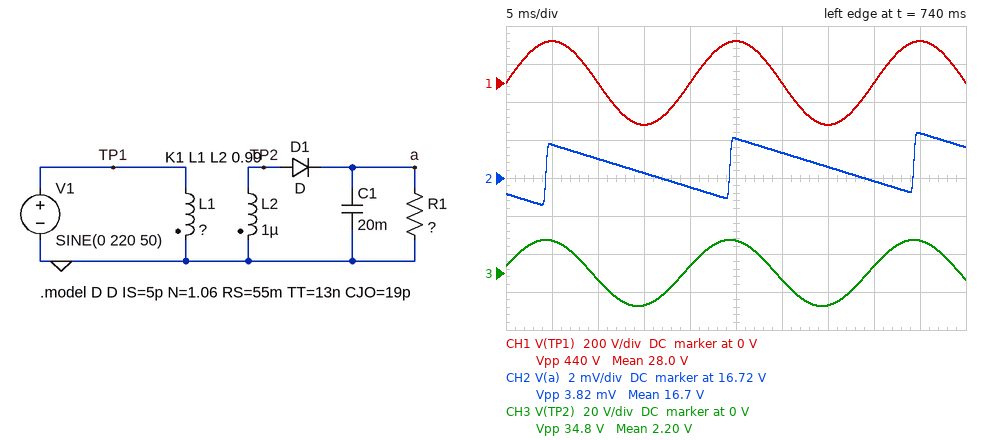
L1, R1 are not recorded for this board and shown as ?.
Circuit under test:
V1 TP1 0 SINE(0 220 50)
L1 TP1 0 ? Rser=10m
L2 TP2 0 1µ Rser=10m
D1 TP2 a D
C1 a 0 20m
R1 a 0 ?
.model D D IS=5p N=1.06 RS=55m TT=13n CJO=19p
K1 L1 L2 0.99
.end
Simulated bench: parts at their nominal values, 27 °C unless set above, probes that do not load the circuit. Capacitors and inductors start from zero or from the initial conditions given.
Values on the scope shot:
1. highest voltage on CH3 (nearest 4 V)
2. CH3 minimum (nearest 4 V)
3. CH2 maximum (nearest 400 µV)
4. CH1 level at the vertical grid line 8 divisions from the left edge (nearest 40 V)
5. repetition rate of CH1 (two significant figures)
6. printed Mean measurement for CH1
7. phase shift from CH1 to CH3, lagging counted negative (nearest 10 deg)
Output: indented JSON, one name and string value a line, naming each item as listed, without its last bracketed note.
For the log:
{
  "highest voltage on CH3": "16 V",
  "CH3 minimum": "-16 V",
  "CH2 maximum": "16.7184 V",
  "CH1 level at the vertical grid line 8 divisions from the left edge": "0 V",
  "repetition rate of CH1": "50 Hz",
  "printed Mean measurement for CH1": "28.0 V",
  "phase shift from CH1 to CH3, lagging counted negative": "10 deg"
}
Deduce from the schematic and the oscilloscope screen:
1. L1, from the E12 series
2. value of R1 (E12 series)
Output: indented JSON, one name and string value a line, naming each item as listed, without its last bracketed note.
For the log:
{
  "L1, from the E12 series": "150 µH",
  "value of R1": "5.6 kΩ"
}
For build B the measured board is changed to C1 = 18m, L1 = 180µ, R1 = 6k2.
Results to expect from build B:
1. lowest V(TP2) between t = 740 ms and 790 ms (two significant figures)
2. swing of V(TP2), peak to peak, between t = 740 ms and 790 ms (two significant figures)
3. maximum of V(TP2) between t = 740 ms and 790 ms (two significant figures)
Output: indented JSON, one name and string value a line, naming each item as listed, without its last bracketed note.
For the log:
{
  "lowest V(TP2) between t = 740 ms and 790 ms": "-16 V",
  "swing of V(TP2), peak to peak, between t = 740 ms and 790 ms": "32 V",
  "maximum of V(TP2) between t = 740 ms and 790 ms": "16 V"
}
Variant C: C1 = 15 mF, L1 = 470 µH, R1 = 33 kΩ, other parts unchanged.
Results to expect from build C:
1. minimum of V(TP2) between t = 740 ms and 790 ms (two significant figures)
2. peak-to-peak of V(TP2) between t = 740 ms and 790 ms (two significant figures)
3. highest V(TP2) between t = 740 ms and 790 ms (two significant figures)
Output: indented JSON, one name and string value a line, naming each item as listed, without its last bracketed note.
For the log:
{
  "minimum of V(TP2) between t = 740 ms and 790 ms": "-10 V",
  "peak-to-peak of V(TP2) between t = 740 ms and 790 ms": "20 V",
  "highest V(TP2) between t = 740 ms and 790 ms": "10 V"
}
